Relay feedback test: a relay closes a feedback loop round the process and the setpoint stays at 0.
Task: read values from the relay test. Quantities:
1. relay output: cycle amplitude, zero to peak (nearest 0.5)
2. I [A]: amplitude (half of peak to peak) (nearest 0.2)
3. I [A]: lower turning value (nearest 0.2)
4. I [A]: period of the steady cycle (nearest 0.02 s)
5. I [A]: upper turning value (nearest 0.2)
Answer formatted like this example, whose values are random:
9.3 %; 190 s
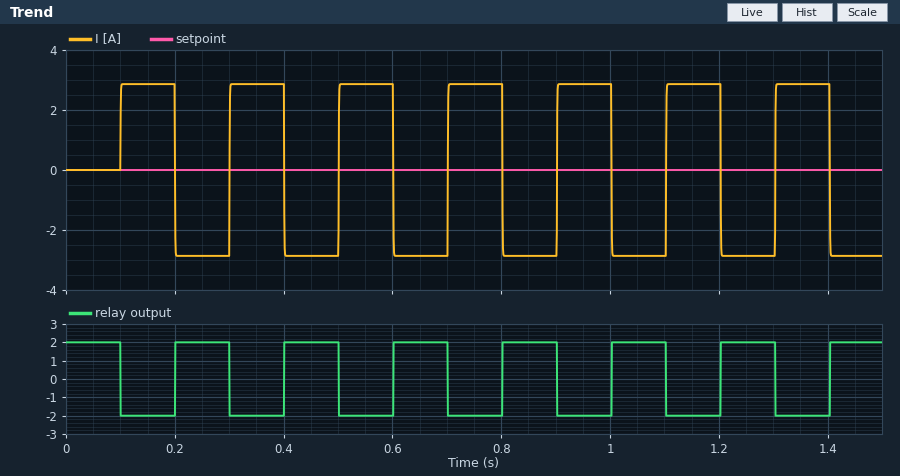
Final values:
2.0; 2.8; -2.8; 0.20 s; 2.8
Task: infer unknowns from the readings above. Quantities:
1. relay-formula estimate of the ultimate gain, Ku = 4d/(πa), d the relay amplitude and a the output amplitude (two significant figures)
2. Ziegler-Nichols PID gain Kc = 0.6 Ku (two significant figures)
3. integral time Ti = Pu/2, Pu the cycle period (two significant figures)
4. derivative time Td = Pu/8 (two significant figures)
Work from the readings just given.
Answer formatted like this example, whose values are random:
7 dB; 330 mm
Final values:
0.91; 0.55; 0.10 s; 0.025 s
